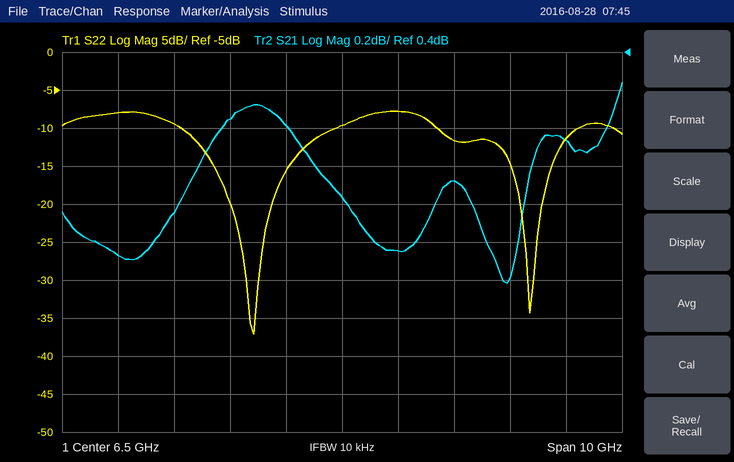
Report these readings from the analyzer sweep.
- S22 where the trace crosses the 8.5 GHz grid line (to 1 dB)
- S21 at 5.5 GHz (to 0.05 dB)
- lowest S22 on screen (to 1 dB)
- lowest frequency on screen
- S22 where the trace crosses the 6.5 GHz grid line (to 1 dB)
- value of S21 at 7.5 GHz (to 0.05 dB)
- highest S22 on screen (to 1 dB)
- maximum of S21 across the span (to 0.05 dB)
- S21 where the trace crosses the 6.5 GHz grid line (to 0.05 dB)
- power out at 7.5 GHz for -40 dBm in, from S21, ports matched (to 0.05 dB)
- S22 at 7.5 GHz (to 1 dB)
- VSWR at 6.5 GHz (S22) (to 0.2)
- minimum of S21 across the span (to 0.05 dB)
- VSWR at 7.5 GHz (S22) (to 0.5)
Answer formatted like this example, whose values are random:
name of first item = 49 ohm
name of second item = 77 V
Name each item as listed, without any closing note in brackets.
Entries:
S22 where the trace crosses the 8.5 GHz grid line = -12 dB
S21 at 5.5 GHz = 0.00 dB
lowest S22 on screen = -37 dB
lowest frequency on screen = 1.5 GHz
S22 where the trace crosses the 6.5 GHz grid line = -10 dB
value of S21 at 7.5 GHz = -0.65 dB
highest S22 on screen = -8 dB
maximum of S21 across the span = 0.25 dB
S21 where the trace crosses the 6.5 GHz grid line = -0.35 dB
power out at 7.5 GHz for -40 dBm in, from S21, ports matched = -40.65 dBm
S22 at 7.5 GHz = -8 dB
VSWR at 6.5 GHz (S22) = 2.0
minimum of S21 across the span = -0.80 dB
VSWR at 7.5 GHz (S22) = 2.5
